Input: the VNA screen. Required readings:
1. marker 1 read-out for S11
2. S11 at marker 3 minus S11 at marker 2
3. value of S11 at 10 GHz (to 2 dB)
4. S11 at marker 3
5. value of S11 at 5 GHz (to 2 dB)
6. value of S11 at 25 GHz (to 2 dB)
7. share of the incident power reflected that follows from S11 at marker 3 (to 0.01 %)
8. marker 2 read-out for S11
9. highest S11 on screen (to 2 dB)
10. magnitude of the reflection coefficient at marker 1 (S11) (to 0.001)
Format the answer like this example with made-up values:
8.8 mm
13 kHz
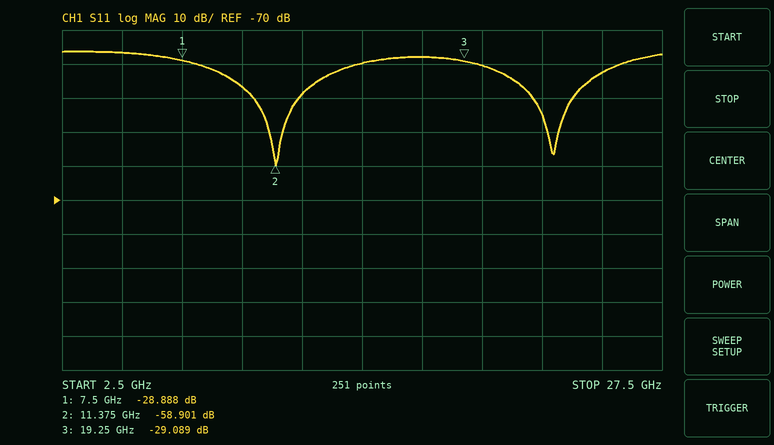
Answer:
-28.888 dB
29.812 dB
-36 dB
-29.089 dB
-26 dB
-32 dB
0.12 %
-58.901 dB
-26 dB
0.036
